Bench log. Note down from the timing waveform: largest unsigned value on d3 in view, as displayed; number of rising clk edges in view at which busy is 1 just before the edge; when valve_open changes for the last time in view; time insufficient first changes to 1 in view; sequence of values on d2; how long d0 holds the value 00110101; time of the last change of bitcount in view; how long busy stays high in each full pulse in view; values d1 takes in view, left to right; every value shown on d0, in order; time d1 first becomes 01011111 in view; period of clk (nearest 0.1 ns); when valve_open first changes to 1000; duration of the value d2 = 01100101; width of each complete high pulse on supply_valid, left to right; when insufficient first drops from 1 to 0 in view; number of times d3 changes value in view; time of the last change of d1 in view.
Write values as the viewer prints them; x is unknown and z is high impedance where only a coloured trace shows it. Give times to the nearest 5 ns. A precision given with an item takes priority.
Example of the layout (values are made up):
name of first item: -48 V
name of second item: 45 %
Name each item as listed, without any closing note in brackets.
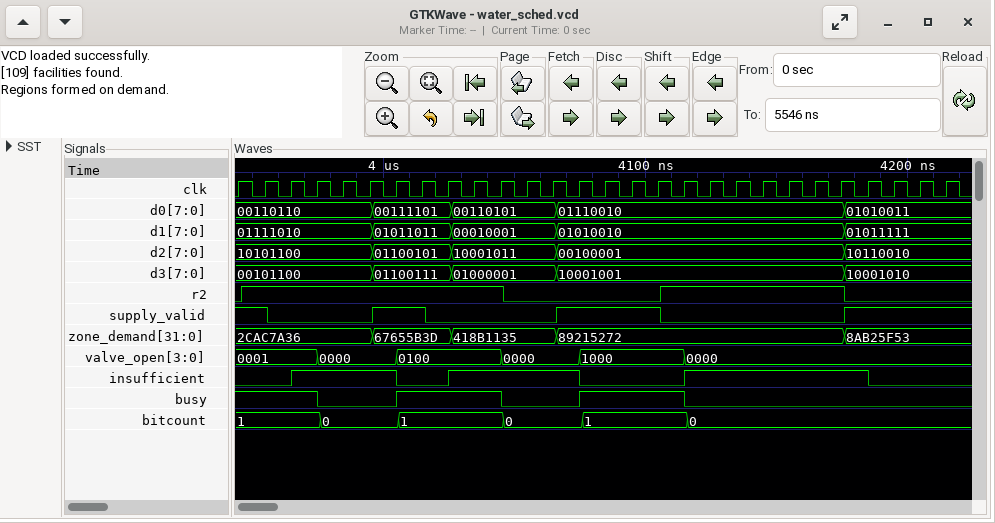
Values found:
largest unsigned value on d3 in view, as displayed: 10001010
number of rising clk edges in view at which busy is 1 just before the edge: 12
when valve_open changes for the last time in view: 4115 ns
time insufficient first changes to 1 in view: 3965 ns
sequence of values on d2: 10101100, 01100101, 10001011, 00100001, 10110010
how long d0 holds the value 00110101: 40 ns
time of the last change of bitcount in view: 4115 ns
how long busy stays high in each full pulse in view: 40 ns, 40 ns
values d1 takes in view, left to right: 01111010, 01011011, 00010001, 01010010, 01011111
every value shown on d0, in order: 00110110, 00111101, 00110101, 01110010, 01010011
time d1 first becomes 01011111 in view: 4175 ns
period of clk: 10 ns
when valve_open first changes to 1000: 4075 ns
duration of the value d2 = 01100101: 30 ns
width of each complete high pulse on supply_valid, left to right: 20 ns, 40 ns
when insufficient first drops from 1 to 0 in view: 4005 ns
number of times d3 changes value in view: 4
time of the last change of d1 in view: 4175 ns
